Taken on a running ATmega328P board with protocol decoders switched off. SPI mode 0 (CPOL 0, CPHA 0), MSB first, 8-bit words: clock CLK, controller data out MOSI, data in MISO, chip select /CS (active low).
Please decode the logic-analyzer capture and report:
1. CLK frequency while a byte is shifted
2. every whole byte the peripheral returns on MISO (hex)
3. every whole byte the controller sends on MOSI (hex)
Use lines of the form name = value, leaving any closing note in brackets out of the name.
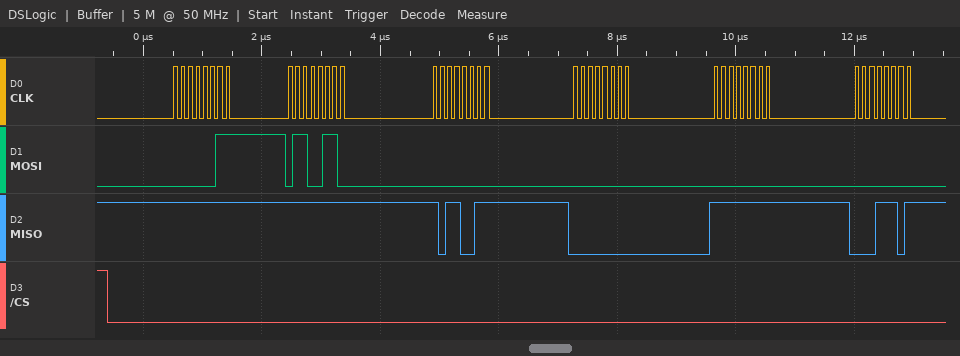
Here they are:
CLK frequency while a byte is shifted = 8 MHz
every whole byte the peripheral returns on MISO = FF FF B3 00 FF 1D
every whole byte the controller sends on MOSI = 03 66 00 00 00 00
